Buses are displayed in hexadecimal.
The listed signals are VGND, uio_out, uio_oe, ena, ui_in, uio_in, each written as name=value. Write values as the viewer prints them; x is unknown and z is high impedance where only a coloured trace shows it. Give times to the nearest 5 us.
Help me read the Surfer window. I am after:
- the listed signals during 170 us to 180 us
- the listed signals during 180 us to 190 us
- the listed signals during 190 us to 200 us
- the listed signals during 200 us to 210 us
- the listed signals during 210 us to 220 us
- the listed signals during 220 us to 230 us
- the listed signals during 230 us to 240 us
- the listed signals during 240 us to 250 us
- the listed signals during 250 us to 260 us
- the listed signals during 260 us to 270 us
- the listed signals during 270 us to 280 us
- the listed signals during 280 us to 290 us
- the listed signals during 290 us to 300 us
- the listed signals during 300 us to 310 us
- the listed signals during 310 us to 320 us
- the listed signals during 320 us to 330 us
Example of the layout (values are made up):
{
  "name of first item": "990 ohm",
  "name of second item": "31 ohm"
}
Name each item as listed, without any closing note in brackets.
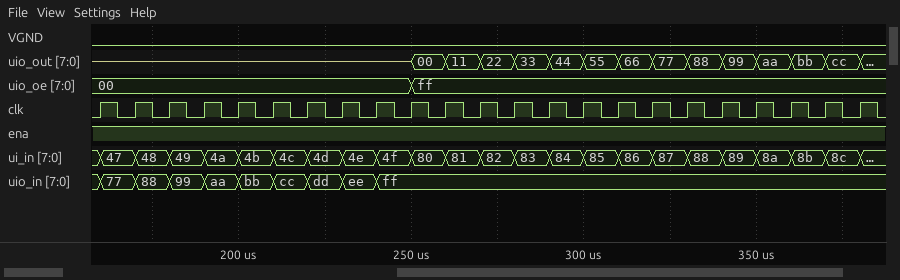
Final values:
{
  "the listed signals during 170 us to 180 us": "VGND=0, uio_out=z, uio_oe=00, ena=1, ui_in=48, uio_in=88",
  "the listed signals during 180 us to 190 us": "VGND=0, uio_out=z, uio_oe=00, ena=1, ui_in=49, uio_in=99",
  "the listed signals during 190 us to 200 us": "VGND=0, uio_out=z, uio_oe=00, ena=1, ui_in=4a, uio_in=aa",
  "the listed signals during 200 us to 210 us": "VGND=0, uio_out=z, uio_oe=00, ena=1, ui_in=4b, uio_in=bb",
  "the listed signals during 210 us to 220 us": "VGND=0, uio_out=z, uio_oe=00, ena=1, ui_in=4c, uio_in=cc",
  "the listed signals during 220 us to 230 us": "VGND=0, uio_out=z, uio_oe=00, ena=1, ui_in=4d, uio_in=dd",
  "the listed signals during 230 us to 240 us": "VGND=0, uio_out=z, uio_oe=00, ena=1, ui_in=4e, uio_in=ee",
  "the listed signals during 240 us to 250 us": "VGND=0, uio_out=z, uio_oe=00, ena=1, ui_in=4f, uio_in=ff",
  "the listed signals during 250 us to 260 us": "VGND=0, uio_out=00, uio_oe=ff, ena=1, ui_in=80, uio_in=ff",
  "the listed signals during 260 us to 270 us": "VGND=0, uio_out=11, uio_oe=ff, ena=1, ui_in=81, uio_in=ff",
  "the listed signals during 270 us to 280 us": "VGND=0, uio_out=22, uio_oe=ff, ena=1, ui_in=82, uio_in=ff",
  "the listed signals during 280 us to 290 us": "VGND=0, uio_out=33, uio_oe=ff, ena=1, ui_in=83, uio_in=ff",
  "the listed signals during 290 us to 300 us": "VGND=0, uio_out=44, uio_oe=ff, ena=1, ui_in=84, uio_in=ff",
  "the listed signals during 300 us to 310 us": "VGND=0, uio_out=55, uio_oe=ff, ena=1, ui_in=85, uio_in=ff",
  "the listed signals during 310 us to 320 us": "VGND=0, uio_out=66, uio_oe=ff, ena=1, ui_in=86, uio_in=ff",
  "the listed signals during 320 us to 330 us": "VGND=0, uio_out=77, uio_oe=ff, ena=1, ui_in=87, uio_in=ff"
}
